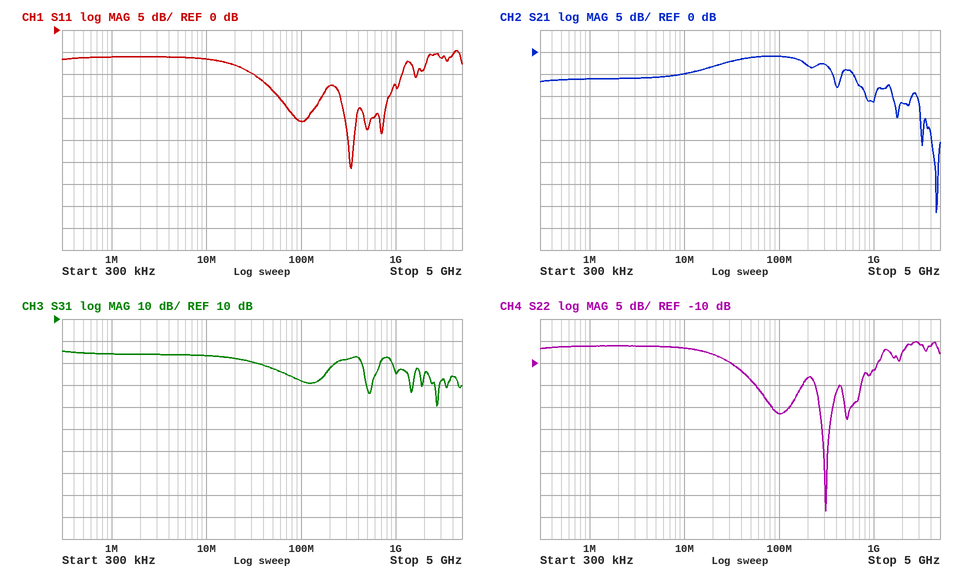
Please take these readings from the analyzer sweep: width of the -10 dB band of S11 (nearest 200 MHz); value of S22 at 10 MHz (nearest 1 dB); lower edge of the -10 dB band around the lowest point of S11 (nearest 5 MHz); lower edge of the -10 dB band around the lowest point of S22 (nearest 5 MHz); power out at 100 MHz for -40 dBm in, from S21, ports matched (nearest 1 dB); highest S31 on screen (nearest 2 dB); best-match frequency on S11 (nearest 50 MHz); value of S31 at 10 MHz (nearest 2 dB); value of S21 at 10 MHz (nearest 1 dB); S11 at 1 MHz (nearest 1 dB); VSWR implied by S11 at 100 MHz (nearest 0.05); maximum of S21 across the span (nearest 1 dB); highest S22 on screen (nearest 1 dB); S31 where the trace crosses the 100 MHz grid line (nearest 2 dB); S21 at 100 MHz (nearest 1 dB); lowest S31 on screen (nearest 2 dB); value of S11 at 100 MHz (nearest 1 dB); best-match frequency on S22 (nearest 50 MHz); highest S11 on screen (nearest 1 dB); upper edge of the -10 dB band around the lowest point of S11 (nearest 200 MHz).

1.2 GHz
-7 dB
30 MHz
30 MHz
-41 dBm
-4 dB
350 MHz
-6 dB
-5 dB
-6 dB
1.20
-1 dB
-5 dB
-18 dB
-1 dB
-30 dB
-21 dB
300 MHz
-5 dB
1.2 GHz
